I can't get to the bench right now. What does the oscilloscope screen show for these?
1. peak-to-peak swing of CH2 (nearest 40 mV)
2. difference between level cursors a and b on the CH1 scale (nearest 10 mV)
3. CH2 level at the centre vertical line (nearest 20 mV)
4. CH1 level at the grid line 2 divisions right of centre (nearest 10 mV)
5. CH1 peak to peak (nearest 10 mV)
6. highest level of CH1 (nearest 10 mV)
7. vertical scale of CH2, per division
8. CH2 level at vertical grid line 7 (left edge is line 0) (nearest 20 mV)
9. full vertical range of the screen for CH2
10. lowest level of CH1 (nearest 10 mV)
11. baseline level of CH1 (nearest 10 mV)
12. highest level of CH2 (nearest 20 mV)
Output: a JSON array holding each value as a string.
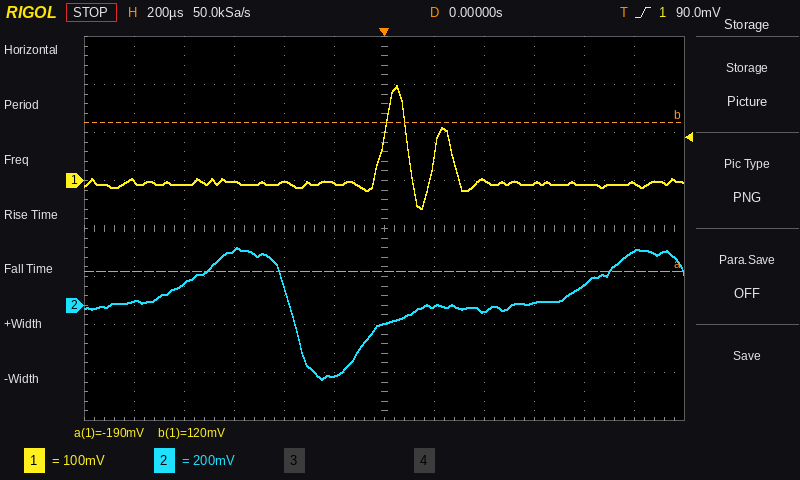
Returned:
["560 mV", "310 mV", "-80 mV", "0 mV", "260 mV", "200 mV", "200 mV", "0 mV", "1.6 V", "-60 mV", "-10 mV", "240 mV"]
